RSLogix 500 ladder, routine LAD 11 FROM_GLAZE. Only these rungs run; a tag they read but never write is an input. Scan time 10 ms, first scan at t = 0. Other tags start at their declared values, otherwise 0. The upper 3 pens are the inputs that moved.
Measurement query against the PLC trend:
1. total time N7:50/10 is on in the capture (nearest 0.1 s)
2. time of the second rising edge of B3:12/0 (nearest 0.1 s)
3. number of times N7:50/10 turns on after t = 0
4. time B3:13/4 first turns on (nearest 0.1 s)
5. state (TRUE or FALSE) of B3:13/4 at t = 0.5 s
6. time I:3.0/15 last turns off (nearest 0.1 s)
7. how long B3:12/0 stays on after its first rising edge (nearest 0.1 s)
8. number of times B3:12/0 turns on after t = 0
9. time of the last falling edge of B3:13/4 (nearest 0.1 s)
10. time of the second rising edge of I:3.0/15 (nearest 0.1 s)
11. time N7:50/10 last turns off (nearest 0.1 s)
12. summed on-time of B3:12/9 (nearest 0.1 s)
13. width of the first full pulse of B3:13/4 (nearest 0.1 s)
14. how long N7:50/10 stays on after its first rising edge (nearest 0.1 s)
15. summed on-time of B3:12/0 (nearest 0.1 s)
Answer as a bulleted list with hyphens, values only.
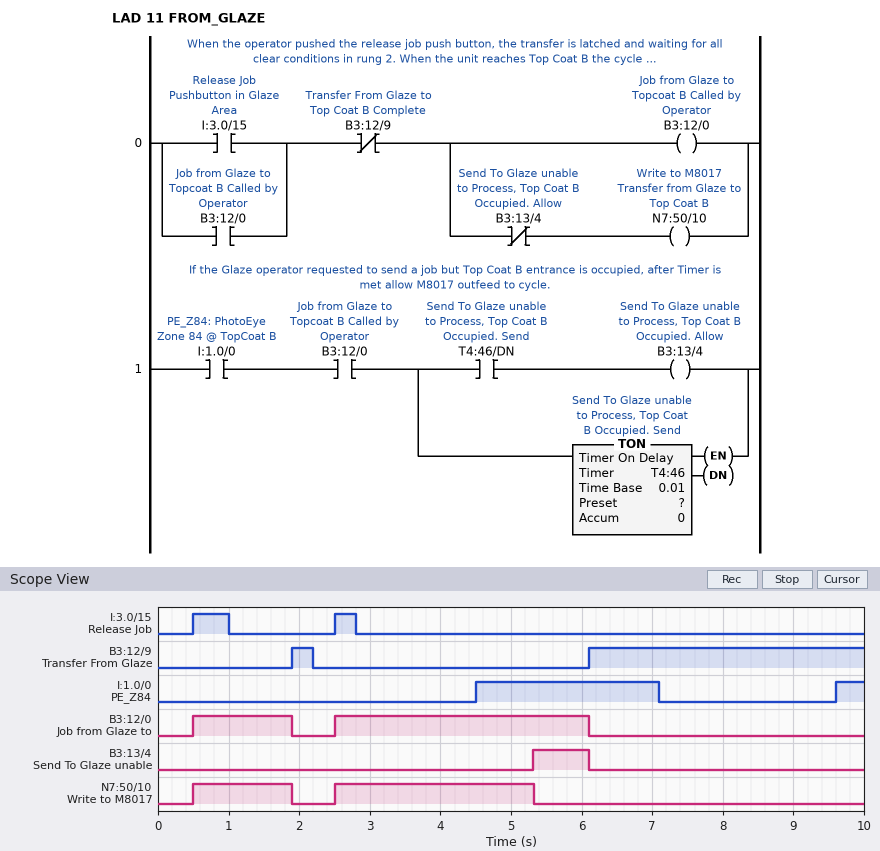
- 4.2 s
- 2.5 s
- 2
- 5.3 s
- FALSE
- 2.8 s
- 1.4 s
- 2
- 6.1 s
- 2.5 s
- 5.3 s
- 4.2 s
- 0.8 s
- 1.4 s
- 5.0 s
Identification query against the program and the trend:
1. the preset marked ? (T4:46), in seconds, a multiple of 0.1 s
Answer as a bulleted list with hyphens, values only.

- 0.8 s
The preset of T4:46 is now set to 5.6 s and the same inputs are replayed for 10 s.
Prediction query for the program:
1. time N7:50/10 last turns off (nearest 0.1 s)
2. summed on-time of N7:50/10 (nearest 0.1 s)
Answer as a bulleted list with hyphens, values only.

- 6.1 s
- 5.0 s
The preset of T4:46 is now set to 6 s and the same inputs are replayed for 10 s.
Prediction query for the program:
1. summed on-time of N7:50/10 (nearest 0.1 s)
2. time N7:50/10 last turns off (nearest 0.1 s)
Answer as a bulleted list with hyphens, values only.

- 5.0 s
- 6.1 s
